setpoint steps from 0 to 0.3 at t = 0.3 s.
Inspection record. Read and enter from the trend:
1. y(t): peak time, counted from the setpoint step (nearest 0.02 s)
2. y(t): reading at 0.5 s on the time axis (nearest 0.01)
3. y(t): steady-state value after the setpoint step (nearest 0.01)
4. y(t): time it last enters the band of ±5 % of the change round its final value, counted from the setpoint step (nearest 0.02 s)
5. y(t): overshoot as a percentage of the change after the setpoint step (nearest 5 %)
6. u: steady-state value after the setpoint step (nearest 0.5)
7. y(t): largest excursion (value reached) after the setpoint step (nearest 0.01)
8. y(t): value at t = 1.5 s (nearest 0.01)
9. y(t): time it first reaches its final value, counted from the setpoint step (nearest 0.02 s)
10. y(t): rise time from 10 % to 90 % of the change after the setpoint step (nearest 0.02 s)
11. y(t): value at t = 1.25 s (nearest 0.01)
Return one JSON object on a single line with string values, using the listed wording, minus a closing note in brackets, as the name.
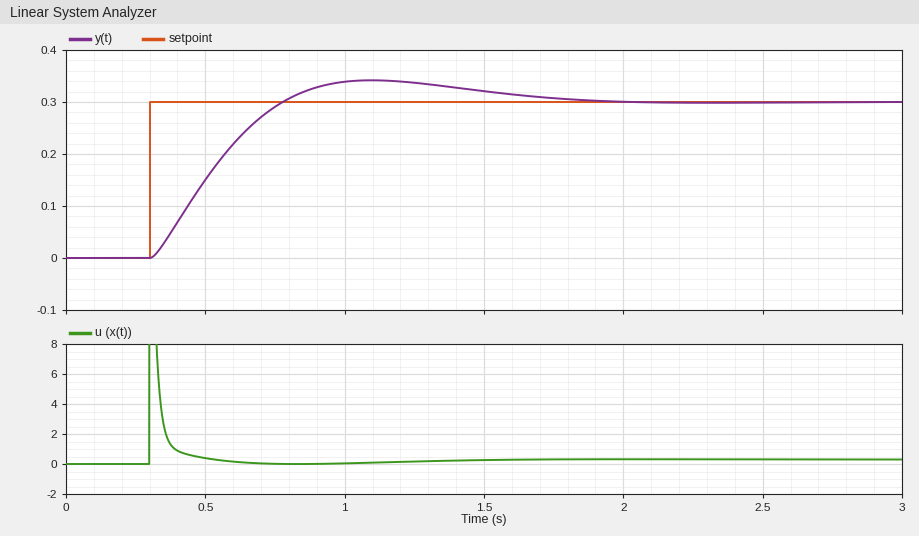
{"y(t): peak time, counted from the setpoint step": "0.80 s", "y(t): reading at 0.5 s on the time axis": "0.15", "y(t): steady-state value after the setpoint step": "0.30", "y(t): time it last enters the band of ±5 % of the change round its final value, counted from the setpoint step": "1.30 s", "y(t): overshoot as a percentage of the change after the setpoint step": "15 %", "u: steady-state value after the setpoint step": "0.5", "y(t): largest excursion (value reached) after the setpoint step": "0.34", "y(t): value at t = 1.5 s": "0.32", "y(t): time it first reaches its final value, counted from the setpoint step": "0.48 s", "y(t): rise time from 10 % to 90 % of the change after the setpoint step": "0.34 s", "y(t): value at t = 1.25 s": "0.34"}
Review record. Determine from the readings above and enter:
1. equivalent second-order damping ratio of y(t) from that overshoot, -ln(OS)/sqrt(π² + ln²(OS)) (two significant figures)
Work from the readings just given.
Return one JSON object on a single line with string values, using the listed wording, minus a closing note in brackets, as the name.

{"equivalent second-order damping ratio of y(t) from that overshoot, -ln(OS)/sqrt(π² + ln²(OS))": "0.52"}
